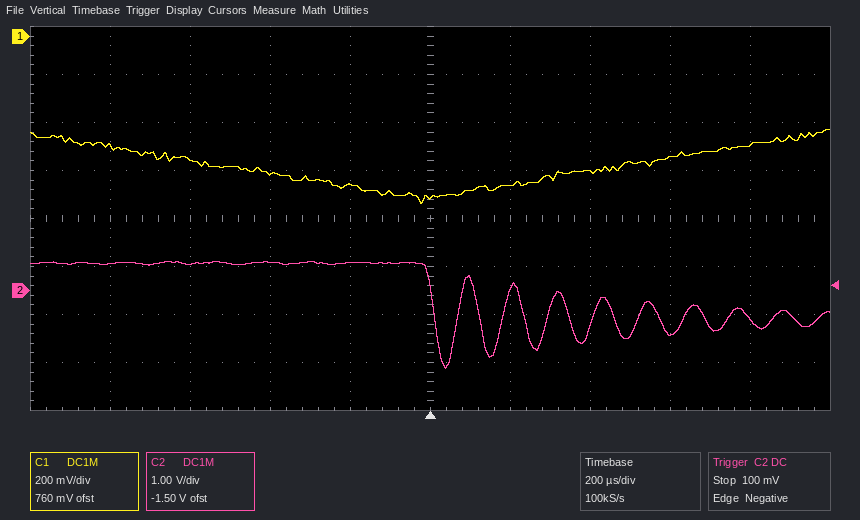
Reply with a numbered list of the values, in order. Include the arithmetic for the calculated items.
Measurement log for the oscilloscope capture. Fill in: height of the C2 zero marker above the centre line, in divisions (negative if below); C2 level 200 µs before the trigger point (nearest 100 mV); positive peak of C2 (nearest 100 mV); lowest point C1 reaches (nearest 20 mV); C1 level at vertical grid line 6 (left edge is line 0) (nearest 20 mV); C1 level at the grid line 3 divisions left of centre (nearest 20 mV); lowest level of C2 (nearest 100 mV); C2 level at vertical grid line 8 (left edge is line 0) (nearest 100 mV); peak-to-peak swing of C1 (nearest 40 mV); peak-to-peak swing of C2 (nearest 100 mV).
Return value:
1. -1.5 div
2. 600 mV
3. 600 mV
4. -700 mV
5. -620 mV
6. -520 mV
7. -1.6 V
8. -900 mV
9. 320 mV
10. 600 mV − (-1.6 V) = 2.2 V
